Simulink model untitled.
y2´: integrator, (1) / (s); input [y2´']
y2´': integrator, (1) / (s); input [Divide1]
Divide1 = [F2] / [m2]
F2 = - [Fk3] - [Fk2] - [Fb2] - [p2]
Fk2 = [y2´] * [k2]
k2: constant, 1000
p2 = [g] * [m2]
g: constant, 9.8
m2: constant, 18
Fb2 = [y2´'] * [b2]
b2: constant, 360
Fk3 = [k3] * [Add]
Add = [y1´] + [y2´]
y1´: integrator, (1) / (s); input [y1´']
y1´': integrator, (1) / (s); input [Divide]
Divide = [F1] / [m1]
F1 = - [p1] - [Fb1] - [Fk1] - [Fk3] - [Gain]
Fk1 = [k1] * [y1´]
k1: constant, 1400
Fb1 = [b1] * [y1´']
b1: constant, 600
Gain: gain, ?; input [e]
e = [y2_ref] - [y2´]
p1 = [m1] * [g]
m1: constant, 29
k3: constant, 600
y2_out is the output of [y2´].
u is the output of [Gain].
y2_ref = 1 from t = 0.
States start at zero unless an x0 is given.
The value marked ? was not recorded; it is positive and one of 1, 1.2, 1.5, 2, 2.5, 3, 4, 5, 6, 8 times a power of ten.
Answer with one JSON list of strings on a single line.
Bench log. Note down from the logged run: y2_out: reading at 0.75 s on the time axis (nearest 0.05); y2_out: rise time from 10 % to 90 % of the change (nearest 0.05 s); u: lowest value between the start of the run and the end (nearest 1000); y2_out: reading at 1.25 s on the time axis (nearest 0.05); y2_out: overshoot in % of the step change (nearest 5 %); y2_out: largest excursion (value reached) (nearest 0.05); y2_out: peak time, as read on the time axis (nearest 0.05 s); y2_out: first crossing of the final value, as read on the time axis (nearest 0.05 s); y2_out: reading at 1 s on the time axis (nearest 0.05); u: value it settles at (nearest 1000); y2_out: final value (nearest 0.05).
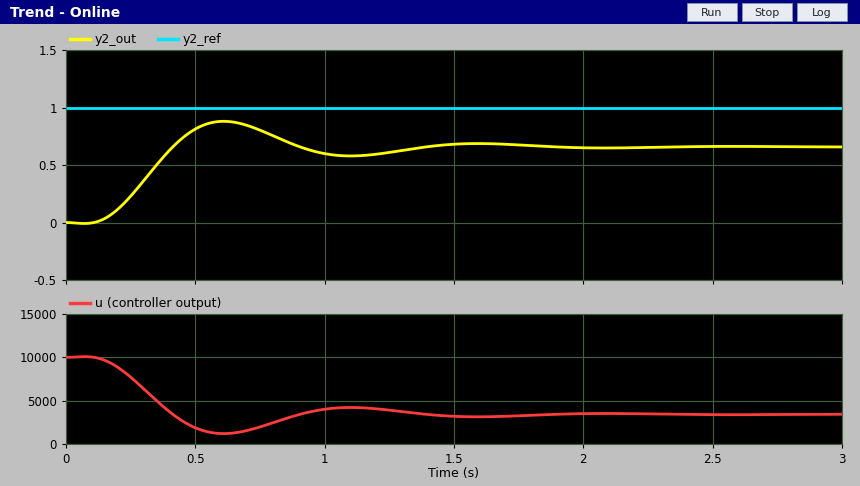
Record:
["0.80", "0.20 s", "1000", "0.60", "35 %", "0.90", "0.60 s", "0.40 s", "0.60", "3000", "0.65"]
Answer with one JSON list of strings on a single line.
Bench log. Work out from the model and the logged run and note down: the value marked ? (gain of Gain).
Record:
["10000"]
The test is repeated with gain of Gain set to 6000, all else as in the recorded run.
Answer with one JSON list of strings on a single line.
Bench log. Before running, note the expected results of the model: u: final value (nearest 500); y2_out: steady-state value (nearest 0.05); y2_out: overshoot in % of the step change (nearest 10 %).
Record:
["3000", "0.55", "20 %"]
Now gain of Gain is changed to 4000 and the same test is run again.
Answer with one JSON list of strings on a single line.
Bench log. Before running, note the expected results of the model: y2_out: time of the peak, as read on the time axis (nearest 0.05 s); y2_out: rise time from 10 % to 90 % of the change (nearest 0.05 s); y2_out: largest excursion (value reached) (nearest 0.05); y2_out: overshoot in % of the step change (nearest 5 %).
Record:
["0.85 s", "0.35 s", "0.45", "10 %"]
